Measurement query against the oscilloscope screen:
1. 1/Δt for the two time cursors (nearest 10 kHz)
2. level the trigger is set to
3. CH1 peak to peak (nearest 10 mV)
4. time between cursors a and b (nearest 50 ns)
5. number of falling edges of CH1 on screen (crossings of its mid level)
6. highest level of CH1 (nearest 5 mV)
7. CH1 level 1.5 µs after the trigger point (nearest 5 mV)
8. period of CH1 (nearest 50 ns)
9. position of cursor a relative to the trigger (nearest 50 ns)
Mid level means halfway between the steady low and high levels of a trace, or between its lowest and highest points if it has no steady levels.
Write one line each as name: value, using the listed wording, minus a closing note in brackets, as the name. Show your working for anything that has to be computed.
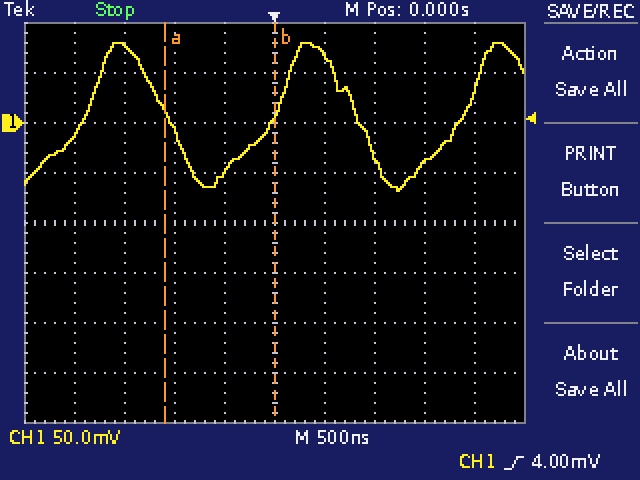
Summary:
1/Δt for the two time cursors: 1 / 1.10 µs ≈ 910 kHz
level the trigger is set to: 4.00 mV
CH1 peak to peak: 150 mV
time between cursors a and b: 1.10 µs
number of falling edges of CH1 on screen: 2
highest level of CH1: 80 mV
CH1 level 1.5 µs after the trigger point: -40 mV
period of CH1: 1.90 µs
position of cursor a relative to the trigger: -1.10 µs
